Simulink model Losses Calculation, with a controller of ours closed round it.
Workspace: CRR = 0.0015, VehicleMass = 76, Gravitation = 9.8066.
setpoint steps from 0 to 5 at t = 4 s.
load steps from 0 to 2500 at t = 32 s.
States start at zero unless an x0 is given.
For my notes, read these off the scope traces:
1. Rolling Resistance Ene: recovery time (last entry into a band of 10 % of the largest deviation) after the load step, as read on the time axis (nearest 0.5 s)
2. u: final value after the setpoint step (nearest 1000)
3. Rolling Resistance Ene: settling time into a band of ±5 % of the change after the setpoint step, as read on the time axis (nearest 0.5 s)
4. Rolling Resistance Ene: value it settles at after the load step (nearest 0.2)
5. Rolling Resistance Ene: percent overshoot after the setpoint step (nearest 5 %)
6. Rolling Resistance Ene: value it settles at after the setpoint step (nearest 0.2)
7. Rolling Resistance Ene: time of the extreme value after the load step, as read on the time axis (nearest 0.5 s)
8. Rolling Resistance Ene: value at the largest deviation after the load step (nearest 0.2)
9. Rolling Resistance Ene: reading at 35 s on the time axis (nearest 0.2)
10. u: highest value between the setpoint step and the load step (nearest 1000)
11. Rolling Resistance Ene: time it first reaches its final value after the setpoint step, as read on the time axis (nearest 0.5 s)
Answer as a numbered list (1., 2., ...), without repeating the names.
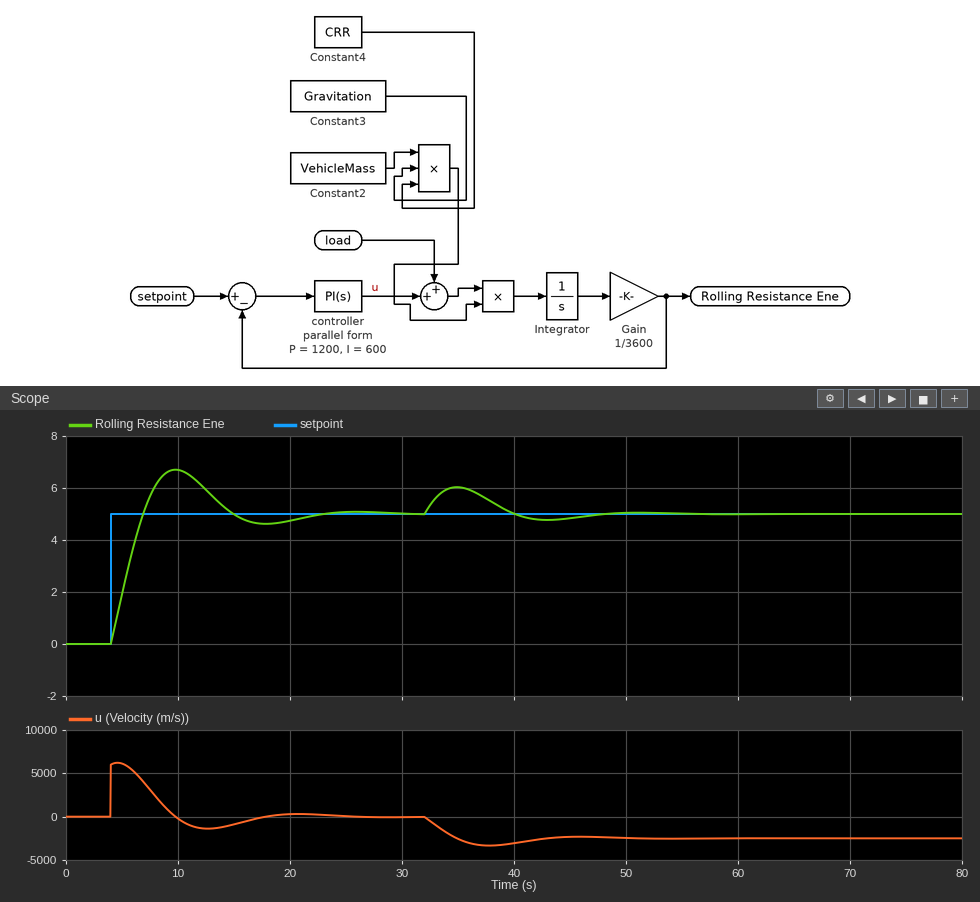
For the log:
1. 46.0 s
2. 0
3. 20.0 s
4. 5.0
5. 35 %
6. 5.0
7. 35.0 s
8. 6.0
9. 6.0
10. 6000
11. 7.0 s
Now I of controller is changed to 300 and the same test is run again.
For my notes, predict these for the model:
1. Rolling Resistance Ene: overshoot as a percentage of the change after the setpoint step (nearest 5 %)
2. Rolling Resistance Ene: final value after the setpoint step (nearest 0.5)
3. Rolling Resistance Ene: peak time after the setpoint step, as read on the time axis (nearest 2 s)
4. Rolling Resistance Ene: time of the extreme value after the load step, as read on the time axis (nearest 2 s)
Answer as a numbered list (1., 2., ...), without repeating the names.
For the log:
1. 25 %
2. 5.0
3. 12 s
4. 36 s
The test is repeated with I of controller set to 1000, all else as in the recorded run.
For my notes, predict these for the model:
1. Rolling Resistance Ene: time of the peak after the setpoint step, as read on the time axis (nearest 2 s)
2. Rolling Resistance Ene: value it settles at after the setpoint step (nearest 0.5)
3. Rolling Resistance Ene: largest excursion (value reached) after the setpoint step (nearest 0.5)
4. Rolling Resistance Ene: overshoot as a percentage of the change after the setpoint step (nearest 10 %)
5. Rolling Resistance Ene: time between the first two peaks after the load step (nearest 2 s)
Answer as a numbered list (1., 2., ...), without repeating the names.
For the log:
1. 8 s
2. 5.0
3. 7.0
4. 40 %
5. 12 s
